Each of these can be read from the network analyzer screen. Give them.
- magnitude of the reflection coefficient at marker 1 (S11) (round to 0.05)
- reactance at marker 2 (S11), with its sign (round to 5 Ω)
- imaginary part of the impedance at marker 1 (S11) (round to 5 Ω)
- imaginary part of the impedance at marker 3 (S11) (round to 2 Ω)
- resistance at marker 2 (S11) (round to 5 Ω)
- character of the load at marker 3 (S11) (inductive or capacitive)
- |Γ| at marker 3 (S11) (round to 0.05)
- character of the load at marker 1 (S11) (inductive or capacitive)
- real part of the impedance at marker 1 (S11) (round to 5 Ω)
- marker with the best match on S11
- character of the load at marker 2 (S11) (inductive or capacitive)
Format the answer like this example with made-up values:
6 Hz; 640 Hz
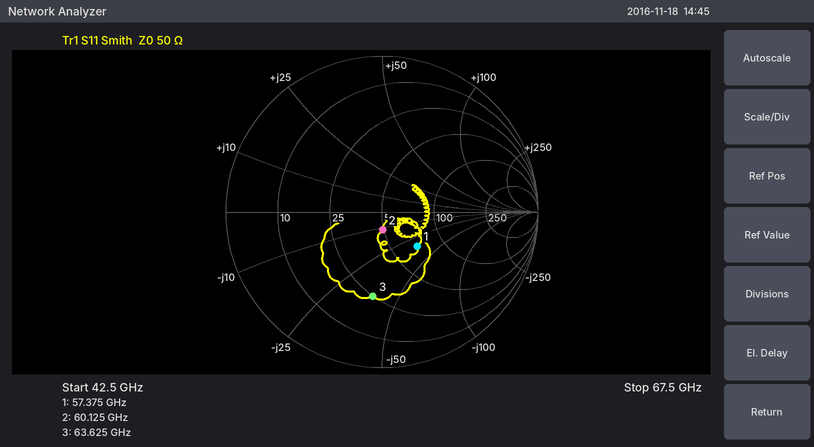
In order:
0.30; -10 Ω; -35 Ω; -38 Ω; 50 Ω; capacitive; 0.55; capacitive; 70 Ω; marker 2; capacitive
